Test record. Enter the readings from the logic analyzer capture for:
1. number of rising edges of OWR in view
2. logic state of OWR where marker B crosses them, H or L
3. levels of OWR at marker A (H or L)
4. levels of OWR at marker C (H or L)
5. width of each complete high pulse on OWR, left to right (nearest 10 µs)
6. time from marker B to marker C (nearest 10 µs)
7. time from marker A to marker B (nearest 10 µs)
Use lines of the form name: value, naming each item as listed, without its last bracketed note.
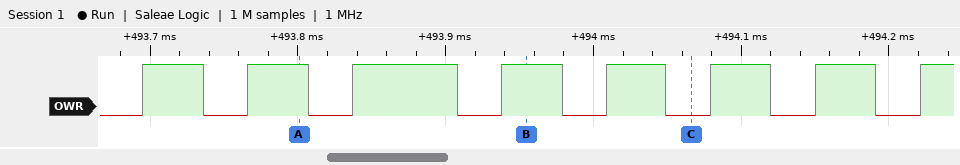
number of rising edges of OWR in view: 8
logic state of OWR where marker B crosses them, H or L: OWR=H
levels of OWR at marker A: OWR=H
levels of OWR at marker C: OWR=L
width of each complete high pulse on OWR, left to right: 40 µs, 40 µs, 70 µs, 40 µs, 40 µs, 40 µs, 40 µs
time from marker B to marker C: 110 µs
time from marker A to marker B: 150 µs
